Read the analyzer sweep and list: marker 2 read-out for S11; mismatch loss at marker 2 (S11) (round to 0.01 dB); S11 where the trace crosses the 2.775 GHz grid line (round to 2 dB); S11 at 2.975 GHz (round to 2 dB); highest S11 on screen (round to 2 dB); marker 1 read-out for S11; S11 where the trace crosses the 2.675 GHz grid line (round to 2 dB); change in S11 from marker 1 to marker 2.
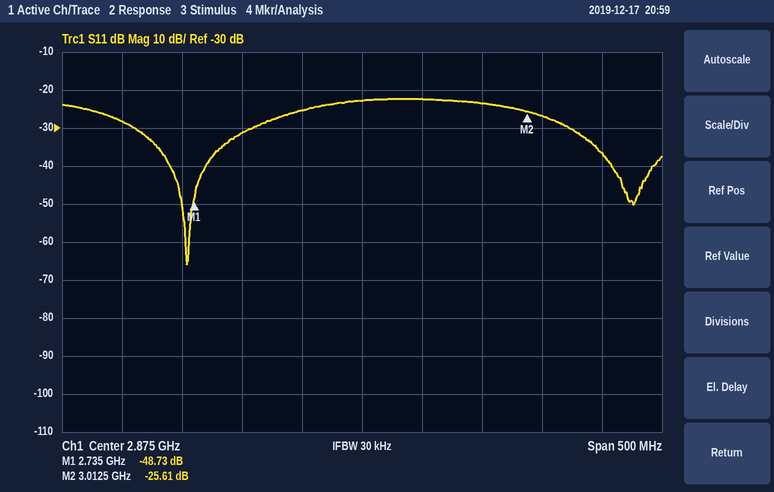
-25.61 dB
0.01 dB
-32 dB
-24 dB
-22 dB
-48.73 dB
-28 dB
23.12 dB
